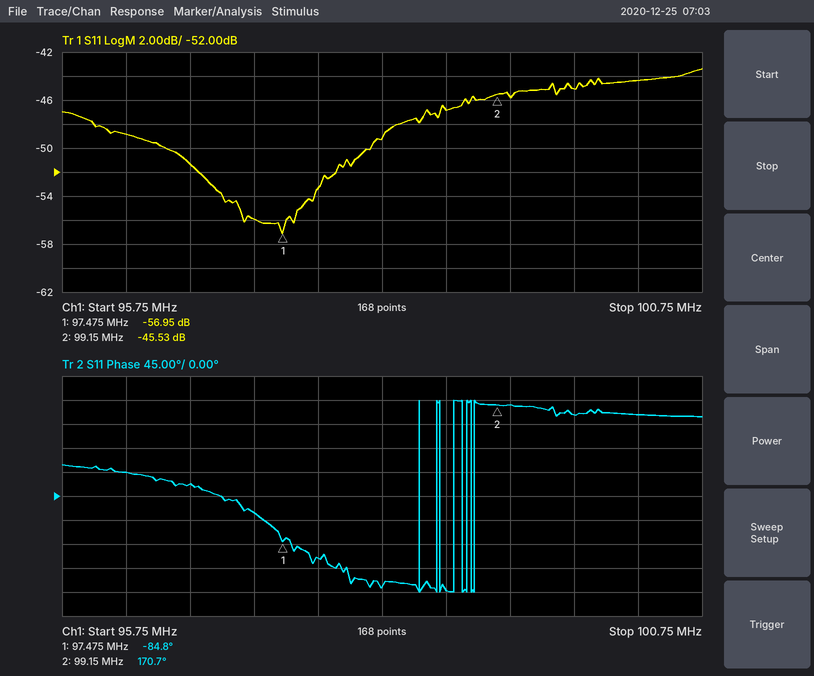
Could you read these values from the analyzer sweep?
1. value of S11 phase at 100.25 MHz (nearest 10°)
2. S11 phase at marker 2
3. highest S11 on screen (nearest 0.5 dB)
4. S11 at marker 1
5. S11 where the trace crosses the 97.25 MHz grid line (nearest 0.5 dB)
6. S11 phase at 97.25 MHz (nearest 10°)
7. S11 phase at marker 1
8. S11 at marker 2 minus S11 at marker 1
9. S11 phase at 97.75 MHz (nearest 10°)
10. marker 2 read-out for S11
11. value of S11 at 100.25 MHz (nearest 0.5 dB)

150°
170.7°
-43.5 dB
-56.95 dB
-56.0 dB
-30°
-84.8°
11.42 dB
-120°
-45.53 dB
-44.5 dB
